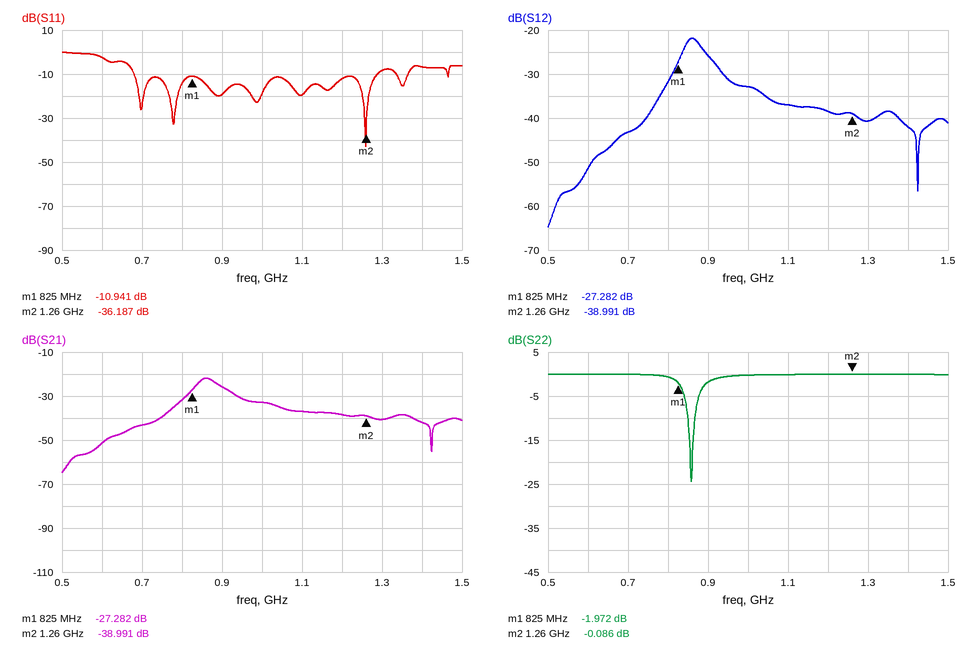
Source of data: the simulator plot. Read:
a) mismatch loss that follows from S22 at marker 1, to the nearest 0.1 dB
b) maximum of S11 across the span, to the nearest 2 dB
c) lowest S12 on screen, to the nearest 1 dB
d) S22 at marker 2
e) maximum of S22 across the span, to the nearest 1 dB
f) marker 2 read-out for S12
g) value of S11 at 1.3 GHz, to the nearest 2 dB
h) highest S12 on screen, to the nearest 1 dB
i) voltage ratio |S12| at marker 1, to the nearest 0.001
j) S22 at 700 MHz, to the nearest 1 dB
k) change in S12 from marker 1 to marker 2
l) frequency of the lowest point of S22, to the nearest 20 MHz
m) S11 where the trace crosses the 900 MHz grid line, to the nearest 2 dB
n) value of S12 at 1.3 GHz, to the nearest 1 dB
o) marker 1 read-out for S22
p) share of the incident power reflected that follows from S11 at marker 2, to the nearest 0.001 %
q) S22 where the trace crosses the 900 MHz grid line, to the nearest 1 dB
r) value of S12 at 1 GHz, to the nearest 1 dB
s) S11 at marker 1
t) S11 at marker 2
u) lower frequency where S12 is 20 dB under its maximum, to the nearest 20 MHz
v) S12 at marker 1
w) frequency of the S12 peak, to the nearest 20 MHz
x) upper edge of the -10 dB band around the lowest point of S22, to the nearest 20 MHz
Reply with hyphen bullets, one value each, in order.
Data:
- 4.4 dB
- 0 dB
- -65 dB
- -0.086 dB
- 0 dB
- -38.991 dB
- -8 dB
- -22 dB
- 0.043
- 0 dB
- -11.709 dB
- 860 MHz
- -20 dB
- -41 dB
- -1.972 dB
- 0.024 %
- -2 dB
- -33 dB
- -10.941 dB
- -36.187 dB
- 720 MHz
- -27.282 dB
- 860 MHz
- 860 MHz
